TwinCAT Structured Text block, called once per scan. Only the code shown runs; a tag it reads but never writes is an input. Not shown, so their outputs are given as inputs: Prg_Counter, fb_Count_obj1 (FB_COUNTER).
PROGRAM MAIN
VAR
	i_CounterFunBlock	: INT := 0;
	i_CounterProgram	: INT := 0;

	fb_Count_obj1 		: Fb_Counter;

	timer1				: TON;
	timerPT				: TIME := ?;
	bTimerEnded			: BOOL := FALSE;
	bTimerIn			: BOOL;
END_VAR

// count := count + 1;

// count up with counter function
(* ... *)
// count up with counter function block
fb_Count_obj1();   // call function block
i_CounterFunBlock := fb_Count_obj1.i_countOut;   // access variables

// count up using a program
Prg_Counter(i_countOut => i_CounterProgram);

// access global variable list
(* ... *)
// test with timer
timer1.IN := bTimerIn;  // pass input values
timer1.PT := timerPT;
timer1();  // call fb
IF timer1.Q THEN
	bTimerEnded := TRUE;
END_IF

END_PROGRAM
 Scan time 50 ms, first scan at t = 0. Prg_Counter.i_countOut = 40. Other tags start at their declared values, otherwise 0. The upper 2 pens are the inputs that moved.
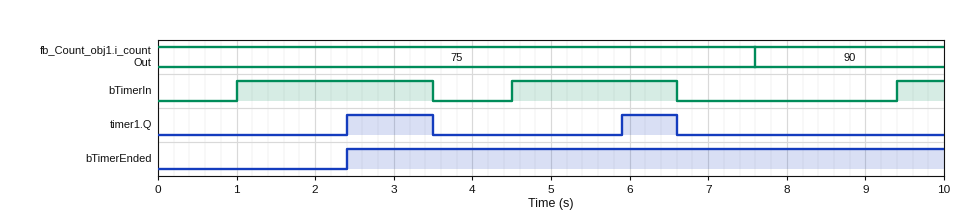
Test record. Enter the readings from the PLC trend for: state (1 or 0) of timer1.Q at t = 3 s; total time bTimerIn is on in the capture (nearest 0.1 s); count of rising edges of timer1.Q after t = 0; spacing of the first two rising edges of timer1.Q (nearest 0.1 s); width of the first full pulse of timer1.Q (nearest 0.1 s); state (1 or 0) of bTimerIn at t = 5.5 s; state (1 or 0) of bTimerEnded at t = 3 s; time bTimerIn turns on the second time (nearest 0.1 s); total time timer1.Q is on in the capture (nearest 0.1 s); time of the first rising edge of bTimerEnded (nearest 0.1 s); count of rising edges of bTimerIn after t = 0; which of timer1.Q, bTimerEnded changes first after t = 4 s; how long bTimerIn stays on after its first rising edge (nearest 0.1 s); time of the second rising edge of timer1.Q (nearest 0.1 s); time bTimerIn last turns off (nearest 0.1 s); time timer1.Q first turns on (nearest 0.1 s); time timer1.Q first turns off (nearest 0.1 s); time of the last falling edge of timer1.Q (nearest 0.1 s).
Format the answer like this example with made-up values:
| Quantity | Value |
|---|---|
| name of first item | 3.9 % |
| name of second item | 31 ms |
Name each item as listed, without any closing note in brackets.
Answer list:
| Quantity | Value |
|---|---|
| state (1 or 0) of timer1.Q at t = 3 s | 1 |
| total time bTimerIn is on in the capture | 5.2 s |
| count of rising edges of timer1.Q after t = 0 | 2 |
| spacing of the first two rising edges of timer1.Q | 3.5 s |
| width of the first full pulse of timer1.Q | 1.1 s |
| state (1 or 0) of bTimerIn at t = 5.5 s | 1 |
| state (1 or 0) of bTimerEnded at t = 3 s | 1 |
| time bTimerIn turns on the second time | 4.5 s |
| total time timer1.Q is on in the capture | 1.8 s |
| time of the first rising edge of bTimerEnded | 2.4 s |
| count of rising edges of bTimerIn after t = 0 | 3 |
| which of timer1.Q, bTimerEnded changes first after t = 4 s | timer1.Q |
| how long bTimerIn stays on after its first rising edge | 2.5 s |
| time of the second rising edge of timer1.Q | 5.9 s |
| time bTimerIn last turns off | 6.6 s |
| time timer1.Q first turns on | 2.4 s |
| time timer1.Q first turns off | 3.5 s |
| time of the last falling edge of timer1.Q | 6.6 s |
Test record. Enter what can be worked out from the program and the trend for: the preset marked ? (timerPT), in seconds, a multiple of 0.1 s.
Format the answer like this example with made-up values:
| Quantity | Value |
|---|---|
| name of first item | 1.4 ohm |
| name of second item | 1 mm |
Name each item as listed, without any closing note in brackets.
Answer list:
| Quantity | Value |
|---|---|
| the preset marked ? (timerPT), in seconds, a multiple of 0.1 s | 1.4 s |
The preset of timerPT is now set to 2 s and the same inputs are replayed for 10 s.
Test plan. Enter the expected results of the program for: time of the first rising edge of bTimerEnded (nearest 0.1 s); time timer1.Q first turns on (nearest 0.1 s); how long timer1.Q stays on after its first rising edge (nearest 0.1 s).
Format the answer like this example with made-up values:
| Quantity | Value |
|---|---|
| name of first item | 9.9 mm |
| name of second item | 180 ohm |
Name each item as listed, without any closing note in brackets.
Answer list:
| Quantity | Value |
|---|---|
| time of the first rising edge of bTimerEnded | 3.0 s |
| time timer1.Q first turns on | 3.0 s |
| how long timer1.Q stays on after its first rising edge | 0.5 s |
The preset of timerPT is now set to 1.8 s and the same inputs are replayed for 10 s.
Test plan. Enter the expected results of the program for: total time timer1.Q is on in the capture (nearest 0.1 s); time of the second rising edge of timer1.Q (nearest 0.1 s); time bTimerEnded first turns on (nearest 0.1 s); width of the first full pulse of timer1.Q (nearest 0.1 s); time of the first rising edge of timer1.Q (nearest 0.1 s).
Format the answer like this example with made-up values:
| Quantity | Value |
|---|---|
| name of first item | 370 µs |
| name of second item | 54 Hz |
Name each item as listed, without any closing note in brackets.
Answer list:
| Quantity | Value |
|---|---|
| total time timer1.Q is on in the capture | 1.0 s |
| time of the second rising edge of timer1.Q | 6.3 s |
| time bTimerEnded first turns on | 2.8 s |
| width of the first full pulse of timer1.Q | 0.7 s |
| time of the first rising edge of timer1.Q | 2.8 s |
